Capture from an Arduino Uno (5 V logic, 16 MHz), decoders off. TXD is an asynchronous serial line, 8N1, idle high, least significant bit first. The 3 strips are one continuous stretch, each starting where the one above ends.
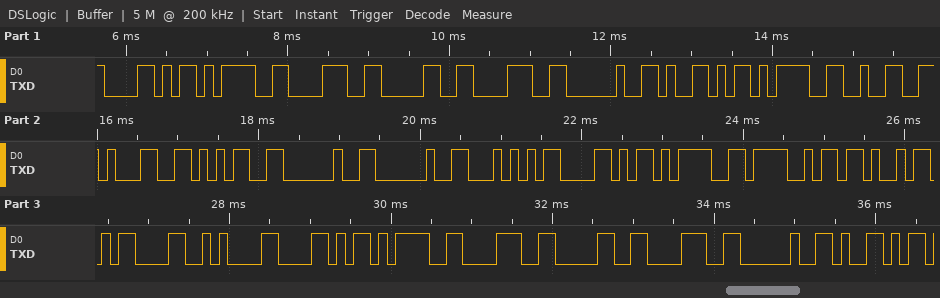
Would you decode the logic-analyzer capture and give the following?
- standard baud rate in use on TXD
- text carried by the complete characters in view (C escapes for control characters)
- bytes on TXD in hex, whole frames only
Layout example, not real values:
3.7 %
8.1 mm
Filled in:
9600 baud
"X=808 Y=215  TX=OK\r\nX=808 Y"
58 3D 38 30 38 20 59 3D 32 31 35 20 20 54 58 3D 4F 4B 0D 0A 58 3D 38 30 38 20 59
